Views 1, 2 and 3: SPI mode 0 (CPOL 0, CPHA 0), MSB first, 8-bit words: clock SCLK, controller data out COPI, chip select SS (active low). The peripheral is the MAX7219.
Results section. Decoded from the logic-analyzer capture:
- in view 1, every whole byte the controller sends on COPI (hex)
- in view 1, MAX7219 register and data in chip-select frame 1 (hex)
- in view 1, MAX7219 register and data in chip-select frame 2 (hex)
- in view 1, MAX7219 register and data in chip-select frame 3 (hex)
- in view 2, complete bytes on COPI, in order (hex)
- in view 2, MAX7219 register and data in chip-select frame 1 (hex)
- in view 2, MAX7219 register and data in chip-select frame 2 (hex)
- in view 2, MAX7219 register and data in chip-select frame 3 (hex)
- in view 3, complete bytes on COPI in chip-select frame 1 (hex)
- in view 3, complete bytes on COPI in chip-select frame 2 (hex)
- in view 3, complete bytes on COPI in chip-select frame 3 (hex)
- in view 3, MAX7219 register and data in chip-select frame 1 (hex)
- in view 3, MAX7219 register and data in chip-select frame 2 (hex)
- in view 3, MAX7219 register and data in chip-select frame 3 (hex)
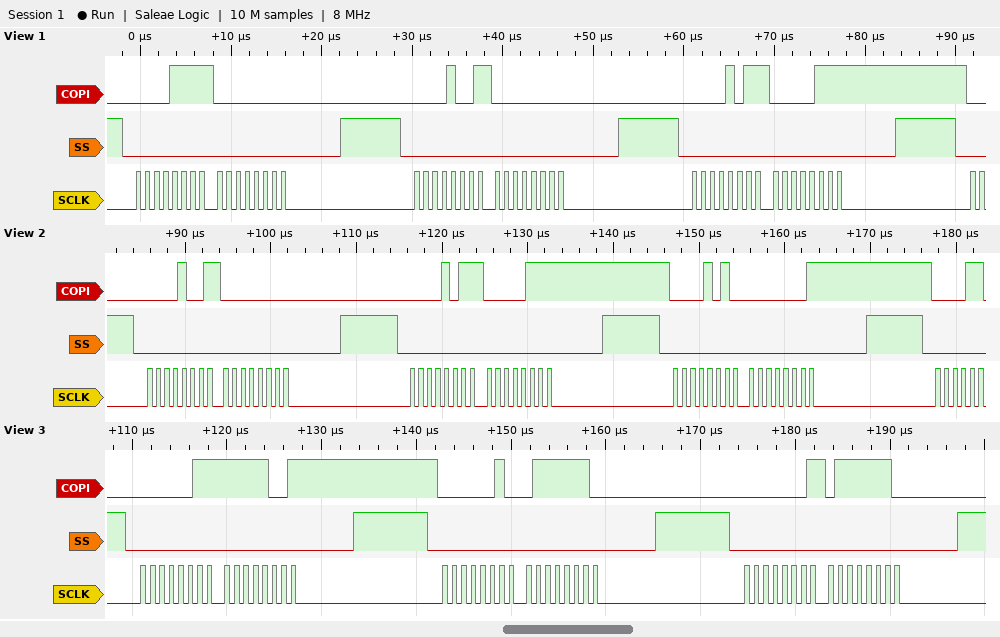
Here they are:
0F 00 09 00 0B 07
register 0xF, data 0x00
register 0x9, data 0x00
register 0xB, data 0x07
0x09 0x00 0x0B 0x07 0x0A 0x01
register 0x9, data 0x00
register 0xB, data 0x07
register 0xA, data 0x01
03 F9
02 7E
01 7E
register 0x3, data 0xF9
register 0x2, data 0x7E
register 0x1, data 0x7E
